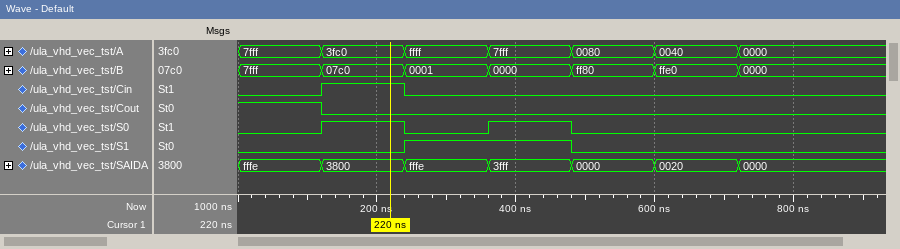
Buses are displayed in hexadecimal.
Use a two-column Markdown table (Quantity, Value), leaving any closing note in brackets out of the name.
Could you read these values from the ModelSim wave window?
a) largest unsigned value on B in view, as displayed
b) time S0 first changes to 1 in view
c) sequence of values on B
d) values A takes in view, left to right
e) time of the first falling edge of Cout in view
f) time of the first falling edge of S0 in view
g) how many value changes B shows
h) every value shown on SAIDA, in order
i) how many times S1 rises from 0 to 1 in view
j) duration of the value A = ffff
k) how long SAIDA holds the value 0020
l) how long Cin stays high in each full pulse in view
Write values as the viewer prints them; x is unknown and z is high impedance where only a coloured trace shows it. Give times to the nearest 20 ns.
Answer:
| Quantity | Value |
|---|---|
| largest unsigned value on B in view, as displayed | ffe0 |
| time S0 first changes to 1 in view | 120 ns |
| sequence of values on B | 7fff, 07c0, 0001, 0000, ff80, ffe0, 0000 |
| values A takes in view, left to right | 7fff, 3fc0, ffff, 7fff, 0080, 0040, 0000 |
| time of the first falling edge of Cout in view | 120 ns |
| time of the first falling edge of S0 in view | 240 ns |
| how many value changes B shows | 6 |
| every value shown on SAIDA, in order | fffe, 3800, fffe, 3fff, 0000, 0020, 0000 |
| how many times S1 rises from 0 to 1 in view | 1 |
| duration of the value A = ffff | 120 ns |
| how long SAIDA holds the value 0020 | 120 ns |
| how long Cin stays high in each full pulse in view | 120 ns |
